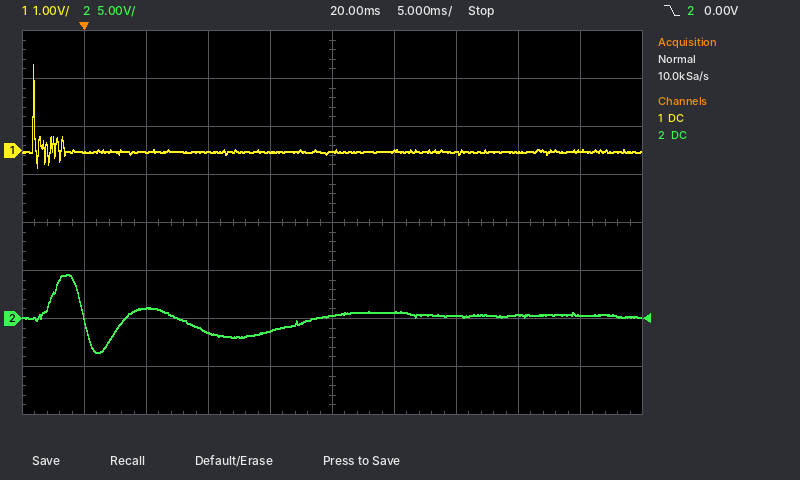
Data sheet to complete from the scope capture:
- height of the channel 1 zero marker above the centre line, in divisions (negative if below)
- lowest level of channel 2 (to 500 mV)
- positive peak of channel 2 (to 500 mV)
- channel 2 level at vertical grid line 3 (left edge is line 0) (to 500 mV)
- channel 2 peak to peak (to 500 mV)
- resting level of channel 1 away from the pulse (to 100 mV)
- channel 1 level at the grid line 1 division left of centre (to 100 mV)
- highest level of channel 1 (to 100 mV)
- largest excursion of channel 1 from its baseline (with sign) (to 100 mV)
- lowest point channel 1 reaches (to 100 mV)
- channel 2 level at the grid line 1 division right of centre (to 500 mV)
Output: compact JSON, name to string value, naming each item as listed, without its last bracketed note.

{"height of the channel 1 zero marker above the centre line, in divisions": "+1.5 div", "lowest level of channel 2": "-3.5 V", "positive peak of channel 2": "4.5 V", "channel 2 level at vertical grid line 3 (left edge is line 0)": "-1.5 V", "channel 2 peak to peak": "8.0 V", "resting level of channel 1 away from the pulse": "0.0 V", "channel 1 level at the grid line 1 division left of centre": "0.0 V", "highest level of channel 1": "1.8 V", "largest excursion of channel 1 from its baseline (with sign)": "+1.8 V", "lowest point channel 1 reaches": "-400 mV", "channel 2 level at the grid line 1 division right of centre": "500 mV"}
